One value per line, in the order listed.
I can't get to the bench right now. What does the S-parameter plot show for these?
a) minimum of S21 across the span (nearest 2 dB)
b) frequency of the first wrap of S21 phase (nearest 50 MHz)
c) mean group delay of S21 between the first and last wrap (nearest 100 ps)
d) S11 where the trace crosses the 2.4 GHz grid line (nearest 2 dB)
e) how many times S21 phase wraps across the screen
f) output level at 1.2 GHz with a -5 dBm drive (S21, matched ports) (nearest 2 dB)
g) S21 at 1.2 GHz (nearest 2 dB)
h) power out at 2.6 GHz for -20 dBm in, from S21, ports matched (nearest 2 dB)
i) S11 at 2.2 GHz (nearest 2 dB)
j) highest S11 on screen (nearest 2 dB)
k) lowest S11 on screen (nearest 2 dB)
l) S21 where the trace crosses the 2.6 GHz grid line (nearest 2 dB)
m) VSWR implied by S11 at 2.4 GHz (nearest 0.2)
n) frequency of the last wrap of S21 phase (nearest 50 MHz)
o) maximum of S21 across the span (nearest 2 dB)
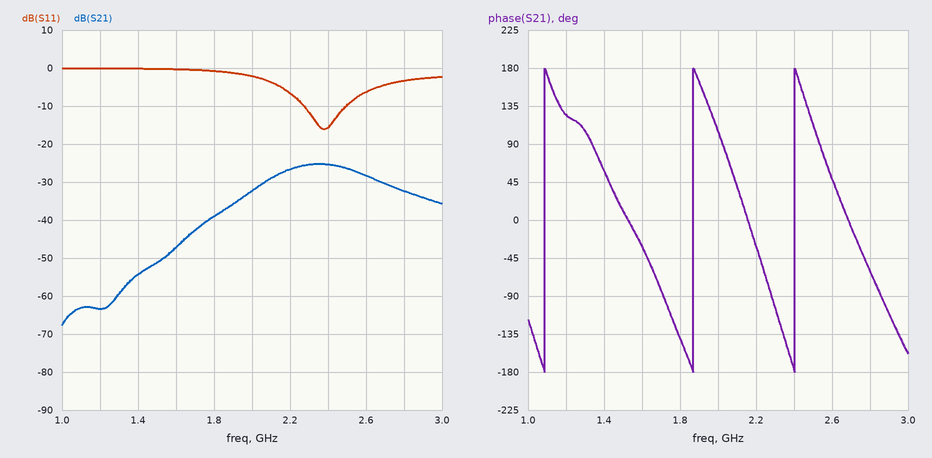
-68 dB
1.10 GHz
1.5 ns
-16 dB
3
-68 dBm
-64 dB
-48 dBm
-6 dB
0 dB
-16 dB
-28 dB
1.4
2.40 GHz
-26 dB
